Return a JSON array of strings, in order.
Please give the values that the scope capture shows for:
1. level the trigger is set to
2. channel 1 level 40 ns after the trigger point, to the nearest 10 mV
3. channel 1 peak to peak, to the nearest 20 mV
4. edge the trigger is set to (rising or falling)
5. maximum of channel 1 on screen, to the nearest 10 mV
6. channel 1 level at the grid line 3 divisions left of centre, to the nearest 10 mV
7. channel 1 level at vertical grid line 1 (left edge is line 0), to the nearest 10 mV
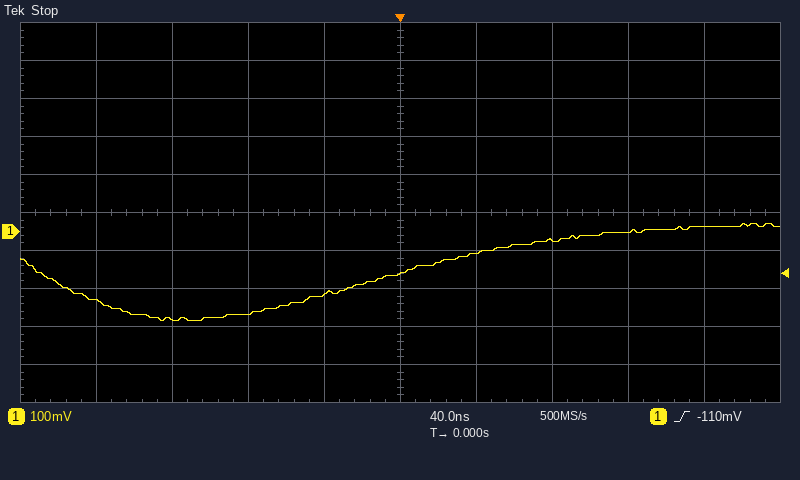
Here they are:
["-110 mV", "-60 mV", "260 mV", "rising", "20 mV", "-230 mV", "-180 mV"]
